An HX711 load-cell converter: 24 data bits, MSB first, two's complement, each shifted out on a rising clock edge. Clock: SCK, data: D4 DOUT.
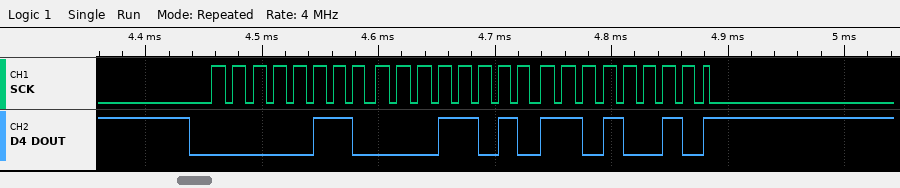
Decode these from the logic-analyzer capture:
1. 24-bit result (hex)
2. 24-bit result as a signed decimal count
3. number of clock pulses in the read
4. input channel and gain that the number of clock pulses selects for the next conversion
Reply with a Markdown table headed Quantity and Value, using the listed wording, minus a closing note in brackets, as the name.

| Quantity | Value |
|---|---|
| 24-bit result | 0x061AD2 |
| 24-bit result as a signed decimal count | 400082 |
| number of clock pulses in the read | 25 |
| input channel and gain that the number of clock pulses selects for the next conversion | channel A, gain 128 |
